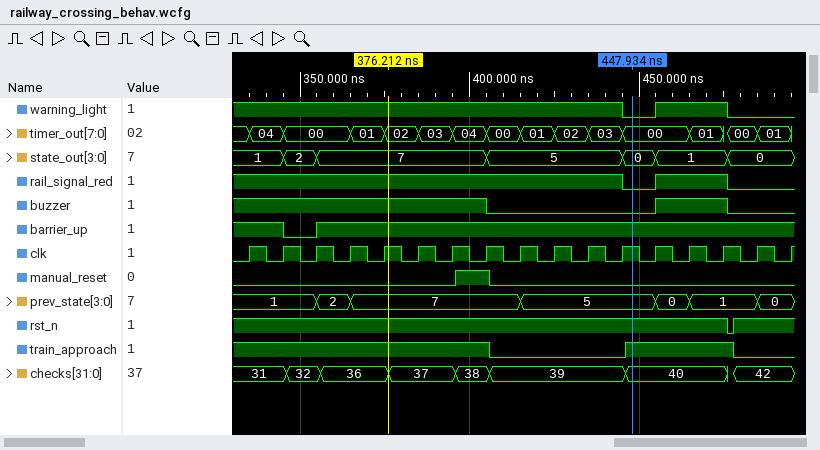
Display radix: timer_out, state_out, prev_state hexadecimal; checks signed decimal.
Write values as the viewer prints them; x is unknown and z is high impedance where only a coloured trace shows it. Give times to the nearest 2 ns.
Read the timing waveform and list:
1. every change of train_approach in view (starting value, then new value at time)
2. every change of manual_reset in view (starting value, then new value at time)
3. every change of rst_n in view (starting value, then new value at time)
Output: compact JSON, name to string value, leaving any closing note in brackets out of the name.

{"every change of train_approach in view": "1, 0 at 406 ns, 1 at 446 ns, 0 at 478 ns", "every change of manual_reset in view": "0, 1 at 396 ns, 0 at 406 ns", "every change of rst_n in view": "1, 0 at 476 ns, 1 at 478 ns"}
